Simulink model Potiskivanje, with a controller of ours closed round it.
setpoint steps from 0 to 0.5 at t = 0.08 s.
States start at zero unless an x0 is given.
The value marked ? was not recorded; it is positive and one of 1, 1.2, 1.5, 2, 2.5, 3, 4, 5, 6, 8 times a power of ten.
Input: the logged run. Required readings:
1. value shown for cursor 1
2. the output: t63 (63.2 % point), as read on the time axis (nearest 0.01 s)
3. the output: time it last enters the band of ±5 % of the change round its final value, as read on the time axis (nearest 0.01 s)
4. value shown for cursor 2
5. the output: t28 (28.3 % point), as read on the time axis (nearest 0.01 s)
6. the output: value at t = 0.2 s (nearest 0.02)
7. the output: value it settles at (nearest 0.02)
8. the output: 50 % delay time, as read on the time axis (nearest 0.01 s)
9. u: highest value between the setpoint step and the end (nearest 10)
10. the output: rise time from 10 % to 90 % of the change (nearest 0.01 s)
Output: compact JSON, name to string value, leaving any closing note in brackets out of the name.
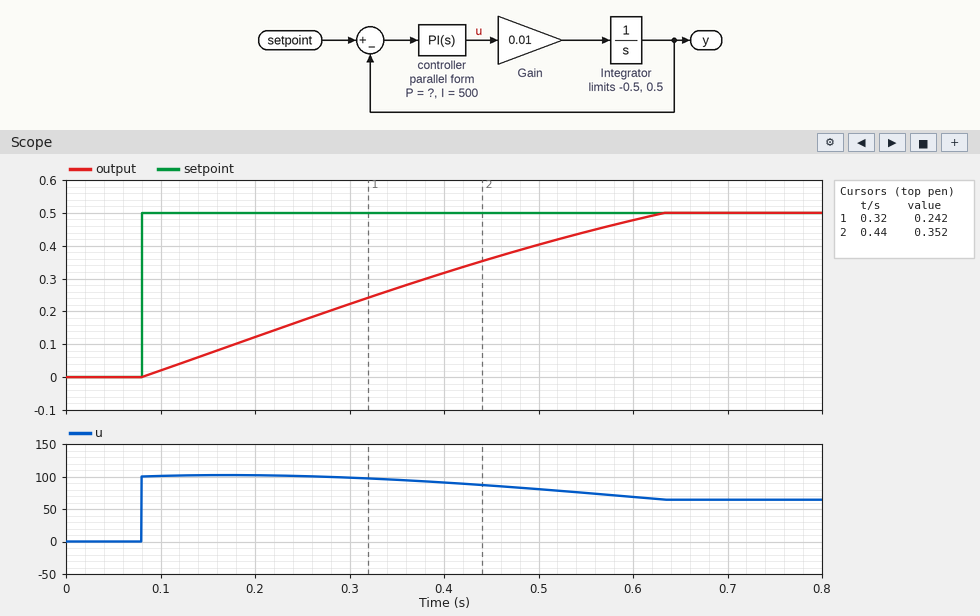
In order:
{"value shown for cursor 1": "0.242", "the output: t63 (63.2 % point), as read on the time axis": "0.40 s", "the output: time it last enters the band of ±5 % of the change round its final value, as read on the time axis": "0.60 s", "value shown for cursor 2": "0.352", "the output: t28 (28.3 % point), as read on the time axis": "0.22 s", "the output: value at t = 0.2 s": "0.12", "the output: value it settles at": "0.50", "the output: 50 % delay time, as read on the time axis": "0.33 s", "u: highest value between the setpoint step and the end": "100", "the output: rise time from 10 % to 90 % of the change": "0.43 s"}
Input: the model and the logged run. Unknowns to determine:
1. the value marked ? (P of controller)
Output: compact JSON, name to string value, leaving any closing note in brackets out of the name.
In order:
{"the value marked ?": "200"}
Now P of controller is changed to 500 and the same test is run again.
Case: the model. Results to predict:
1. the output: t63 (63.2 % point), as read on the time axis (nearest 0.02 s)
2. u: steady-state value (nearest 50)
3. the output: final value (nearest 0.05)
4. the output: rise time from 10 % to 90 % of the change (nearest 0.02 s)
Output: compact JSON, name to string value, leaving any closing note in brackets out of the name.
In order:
{"the output: t63 (63.2 % point), as read on the time axis": "0.26 s", "u: steady-state value": "50", "the output: final value": "0.50", "the output: rise time from 10 % to 90 % of the change": "0.30 s"}
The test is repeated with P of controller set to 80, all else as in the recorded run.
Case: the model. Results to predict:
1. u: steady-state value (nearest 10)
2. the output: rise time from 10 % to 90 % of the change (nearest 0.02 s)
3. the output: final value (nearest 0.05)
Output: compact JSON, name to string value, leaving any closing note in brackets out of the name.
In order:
{"u: steady-state value": "90", "the output: rise time from 10 % to 90 % of the change": "0.48 s", "the output: final value": "0.50"}
